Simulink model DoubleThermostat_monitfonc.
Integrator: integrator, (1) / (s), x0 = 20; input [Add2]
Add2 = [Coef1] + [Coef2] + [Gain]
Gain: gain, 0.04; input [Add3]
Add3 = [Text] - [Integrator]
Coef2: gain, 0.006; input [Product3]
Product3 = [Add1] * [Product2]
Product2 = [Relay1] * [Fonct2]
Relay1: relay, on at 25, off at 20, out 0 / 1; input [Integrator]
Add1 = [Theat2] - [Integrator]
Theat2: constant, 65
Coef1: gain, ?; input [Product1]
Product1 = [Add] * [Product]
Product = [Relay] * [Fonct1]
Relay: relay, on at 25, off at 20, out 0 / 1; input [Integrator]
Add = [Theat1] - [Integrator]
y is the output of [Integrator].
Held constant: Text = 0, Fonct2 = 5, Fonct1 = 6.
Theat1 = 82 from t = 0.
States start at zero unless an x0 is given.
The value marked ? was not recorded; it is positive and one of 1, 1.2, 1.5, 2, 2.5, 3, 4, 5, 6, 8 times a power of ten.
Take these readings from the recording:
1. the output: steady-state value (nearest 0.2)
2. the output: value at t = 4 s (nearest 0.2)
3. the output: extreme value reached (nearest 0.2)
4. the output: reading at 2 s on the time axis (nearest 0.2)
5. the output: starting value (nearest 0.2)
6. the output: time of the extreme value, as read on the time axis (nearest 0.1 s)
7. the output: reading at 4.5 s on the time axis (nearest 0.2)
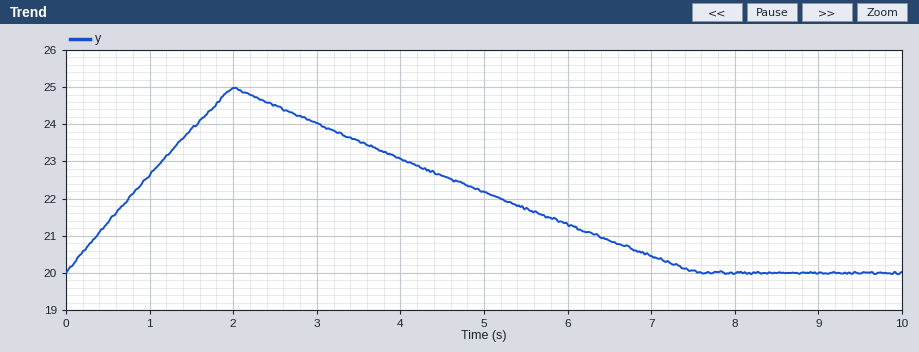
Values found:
20.0
23.0
25.0
25.0
20.0
2.0 s
22.6
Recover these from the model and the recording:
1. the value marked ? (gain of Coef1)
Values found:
0.006
